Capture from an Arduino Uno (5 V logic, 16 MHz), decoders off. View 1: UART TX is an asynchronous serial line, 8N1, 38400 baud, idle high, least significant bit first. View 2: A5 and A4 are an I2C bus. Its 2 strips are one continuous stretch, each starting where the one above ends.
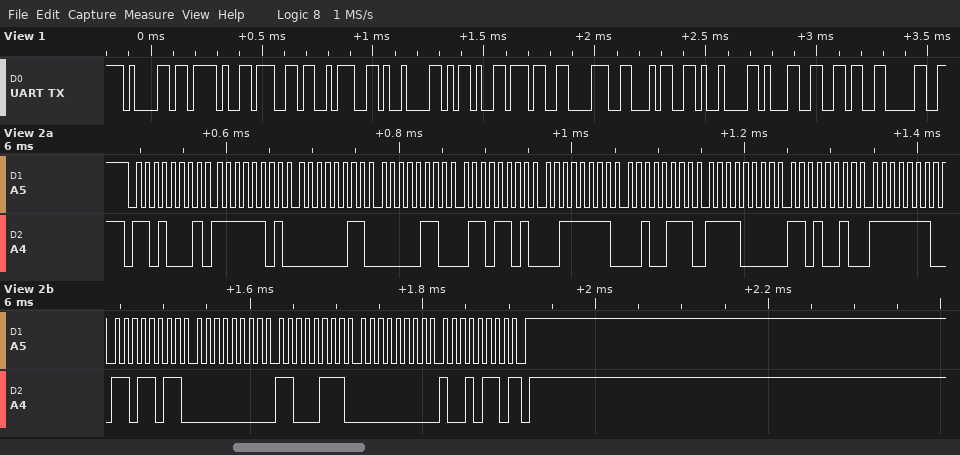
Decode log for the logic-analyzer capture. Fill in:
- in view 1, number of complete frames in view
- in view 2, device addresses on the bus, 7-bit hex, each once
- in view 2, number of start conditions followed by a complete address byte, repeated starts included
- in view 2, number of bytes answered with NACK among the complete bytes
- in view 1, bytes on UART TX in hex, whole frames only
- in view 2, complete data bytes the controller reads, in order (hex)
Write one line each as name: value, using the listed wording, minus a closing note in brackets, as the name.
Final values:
in view 1, number of complete frames in view: 13
in view 2, device addresses on the bus, 7-bit hex, each once: 0x68
in view 2, number of start conditions followed by a complete address byte, repeated starts included: 1
in view 2, number of bytes answered with NACK among the complete bytes: 1
in view 1, bytes on UART TX in hex, whole frames only: 0x61 0x2F 0x67 0x3A 0x09 0x2D 0x37 0x38 0x34 0x09 0x31 0x36 0x30
in view 2, complete data bytes the controller reads, in order: FD 03 06 6D 3F 27 F0 D2 FE DB 00 C7 00 96
